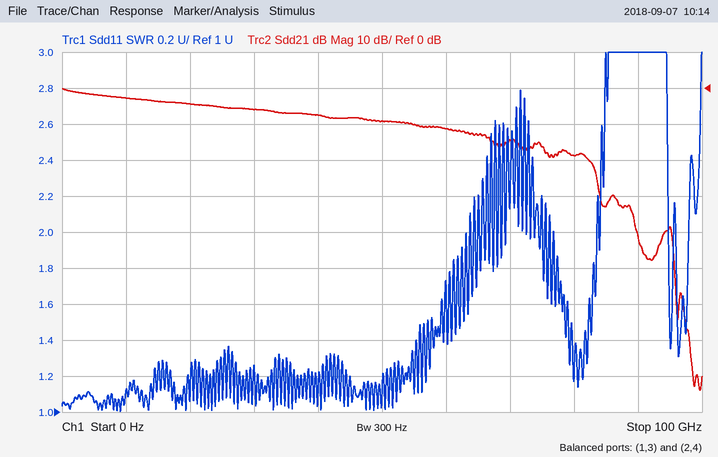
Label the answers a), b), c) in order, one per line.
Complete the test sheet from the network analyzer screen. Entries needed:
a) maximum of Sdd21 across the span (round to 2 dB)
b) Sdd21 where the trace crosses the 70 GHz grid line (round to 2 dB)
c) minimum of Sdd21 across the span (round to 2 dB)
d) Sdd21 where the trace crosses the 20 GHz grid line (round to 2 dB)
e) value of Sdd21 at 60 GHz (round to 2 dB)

a) 0 dB
b) -14 dB
c) -84 dB
d) -4 dB
e) -12 dB
